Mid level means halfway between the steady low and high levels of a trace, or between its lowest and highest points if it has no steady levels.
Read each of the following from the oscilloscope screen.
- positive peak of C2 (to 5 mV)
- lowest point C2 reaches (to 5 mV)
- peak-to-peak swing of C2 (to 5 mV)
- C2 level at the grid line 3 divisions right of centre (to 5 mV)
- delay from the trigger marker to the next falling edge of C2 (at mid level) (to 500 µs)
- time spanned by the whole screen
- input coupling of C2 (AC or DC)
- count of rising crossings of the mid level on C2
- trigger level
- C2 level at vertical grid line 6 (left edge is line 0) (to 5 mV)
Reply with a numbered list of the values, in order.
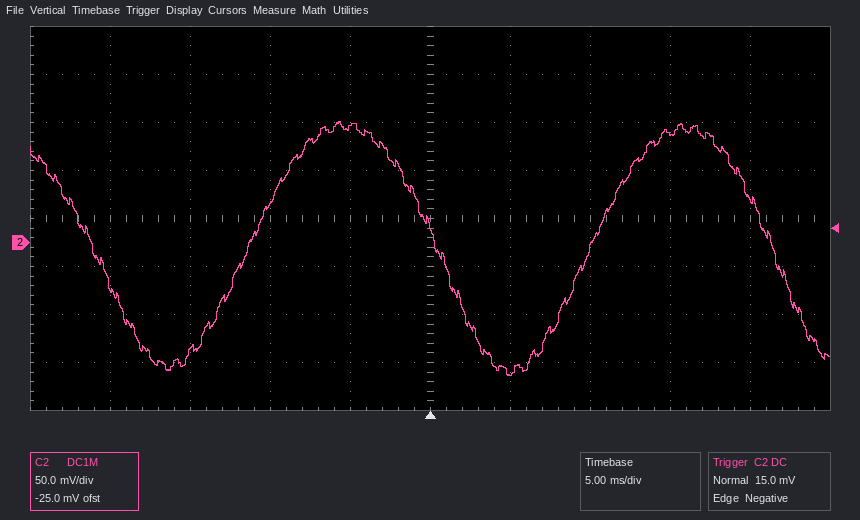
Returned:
1. 125 mV
2. -140 mV
3. 265 mV
4. 115 mV
5. 500 µs
6. 50 ms
7. DC
8. 2
9. 15.0 mV
10. -135 mV
